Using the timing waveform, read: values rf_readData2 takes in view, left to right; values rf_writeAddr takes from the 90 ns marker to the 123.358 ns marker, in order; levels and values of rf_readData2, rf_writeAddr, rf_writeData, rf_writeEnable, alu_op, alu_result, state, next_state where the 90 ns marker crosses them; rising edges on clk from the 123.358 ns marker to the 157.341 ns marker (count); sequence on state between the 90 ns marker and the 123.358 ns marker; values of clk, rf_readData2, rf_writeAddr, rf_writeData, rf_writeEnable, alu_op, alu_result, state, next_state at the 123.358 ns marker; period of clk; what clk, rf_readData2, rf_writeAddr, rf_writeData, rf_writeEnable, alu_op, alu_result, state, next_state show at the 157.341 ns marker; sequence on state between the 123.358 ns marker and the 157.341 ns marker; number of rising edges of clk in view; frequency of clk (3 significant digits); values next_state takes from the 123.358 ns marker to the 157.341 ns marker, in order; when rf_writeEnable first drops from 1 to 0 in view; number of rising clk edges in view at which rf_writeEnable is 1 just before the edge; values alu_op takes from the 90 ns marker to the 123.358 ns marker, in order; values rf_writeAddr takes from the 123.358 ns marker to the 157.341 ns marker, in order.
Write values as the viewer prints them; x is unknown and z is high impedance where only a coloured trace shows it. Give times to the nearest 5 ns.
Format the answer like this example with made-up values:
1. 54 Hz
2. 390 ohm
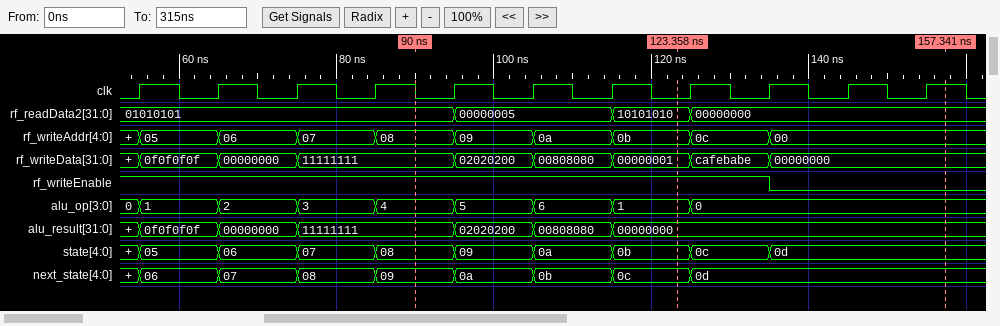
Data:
1. 01010101, 00000005, 10101010, 00000000
2. 08, 09, 0a, 0b
3. rf_readData2=01010101, rf_writeAddr=08, rf_writeData=11111111, rf_writeEnable=1, alu_op=4, alu_result=11111111, state=08, next_state=09
4. 4
5. 08, 09, 0a, 0b
6. clk=0, rf_readData2=10101010, rf_writeAddr=0b, rf_writeData=00000001, rf_writeEnable=1, alu_op=1, alu_result=00000000, state=0b, next_state=0c
7. 10 ns
8. clk=1, rf_readData2=00000000, rf_writeAddr=00, rf_writeData=00000000, rf_writeEnable=0, alu_op=0, alu_result=00000000, state=0d, next_state=0d
9. 0b, 0c, 0d
10. 11
11. 100 MHz
12. 0c, 0d
13. 135 ns
14. 9
15. 4, 5, 6, 1
16. 0b, 0c, 00
